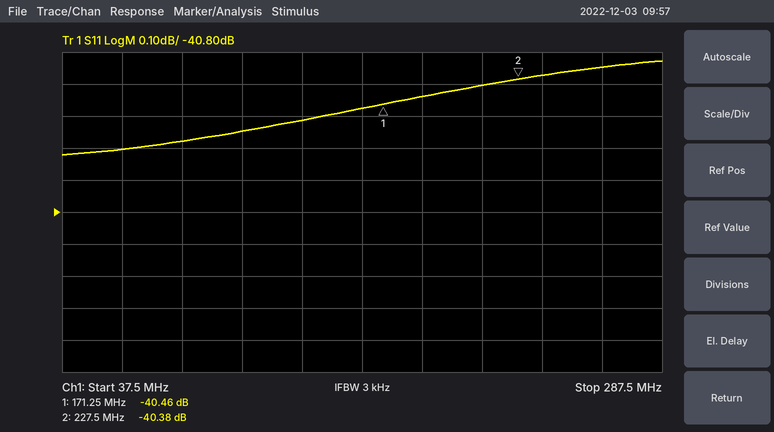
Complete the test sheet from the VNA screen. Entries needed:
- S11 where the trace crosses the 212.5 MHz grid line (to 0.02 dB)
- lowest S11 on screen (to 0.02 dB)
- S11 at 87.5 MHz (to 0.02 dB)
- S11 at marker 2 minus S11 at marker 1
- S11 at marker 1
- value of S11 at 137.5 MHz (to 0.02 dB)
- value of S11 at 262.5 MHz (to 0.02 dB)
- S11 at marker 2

-40.40 dB
-40.62 dB
-40.58 dB
0.08 dB
-40.46 dB
-40.52 dB
-40.34 dB
-40.38 dB
